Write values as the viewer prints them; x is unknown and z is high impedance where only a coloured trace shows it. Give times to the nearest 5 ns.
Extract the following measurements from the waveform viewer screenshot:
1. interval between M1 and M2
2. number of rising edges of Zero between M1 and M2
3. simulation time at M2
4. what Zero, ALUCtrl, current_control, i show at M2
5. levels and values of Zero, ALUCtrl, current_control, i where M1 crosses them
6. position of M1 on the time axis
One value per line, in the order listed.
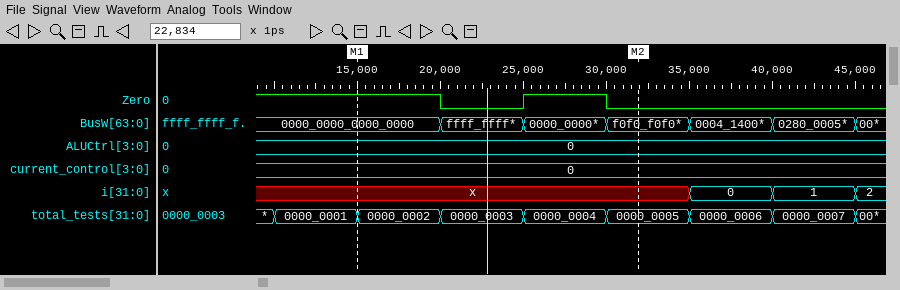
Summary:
15 ns
1
30 ns
Zero=0, ALUCtrl=0, current_control=0, i=x
Zero=1, ALUCtrl=0, current_control=0, i=x
15 ns
